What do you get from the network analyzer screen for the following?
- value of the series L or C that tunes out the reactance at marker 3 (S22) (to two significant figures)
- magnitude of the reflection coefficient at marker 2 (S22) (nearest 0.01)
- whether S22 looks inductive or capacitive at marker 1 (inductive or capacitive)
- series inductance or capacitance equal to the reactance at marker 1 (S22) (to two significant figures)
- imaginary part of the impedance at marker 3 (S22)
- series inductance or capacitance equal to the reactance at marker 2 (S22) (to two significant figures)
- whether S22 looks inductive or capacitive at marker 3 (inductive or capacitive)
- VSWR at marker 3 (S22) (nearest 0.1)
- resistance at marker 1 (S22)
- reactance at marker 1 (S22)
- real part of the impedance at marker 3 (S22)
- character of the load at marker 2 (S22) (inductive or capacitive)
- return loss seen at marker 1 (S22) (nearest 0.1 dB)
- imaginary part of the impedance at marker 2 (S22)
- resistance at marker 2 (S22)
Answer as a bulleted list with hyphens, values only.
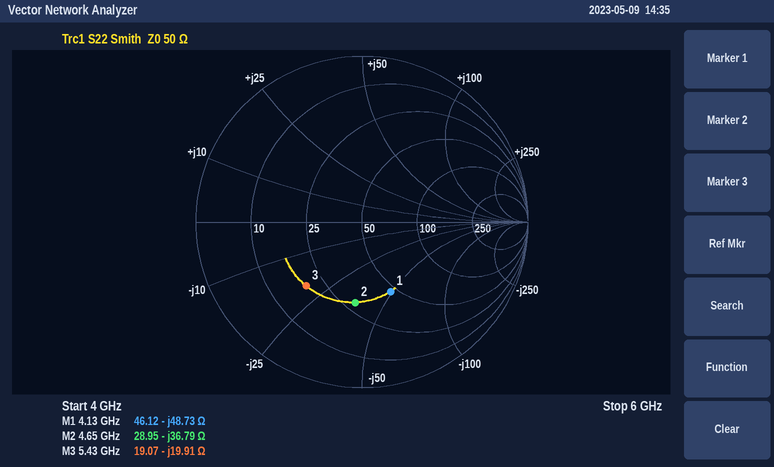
- 580 pH
- 0.49
- capacitive
- 790 fF
- -19.91 Ω
- 930 fF
- capacitive
- 3.1
- 46.12 Ω
- -48.73 Ω
- 19.07 Ω
- capacitive
- 6.9 dB
- -36.79 Ω
- 28.95 Ω
